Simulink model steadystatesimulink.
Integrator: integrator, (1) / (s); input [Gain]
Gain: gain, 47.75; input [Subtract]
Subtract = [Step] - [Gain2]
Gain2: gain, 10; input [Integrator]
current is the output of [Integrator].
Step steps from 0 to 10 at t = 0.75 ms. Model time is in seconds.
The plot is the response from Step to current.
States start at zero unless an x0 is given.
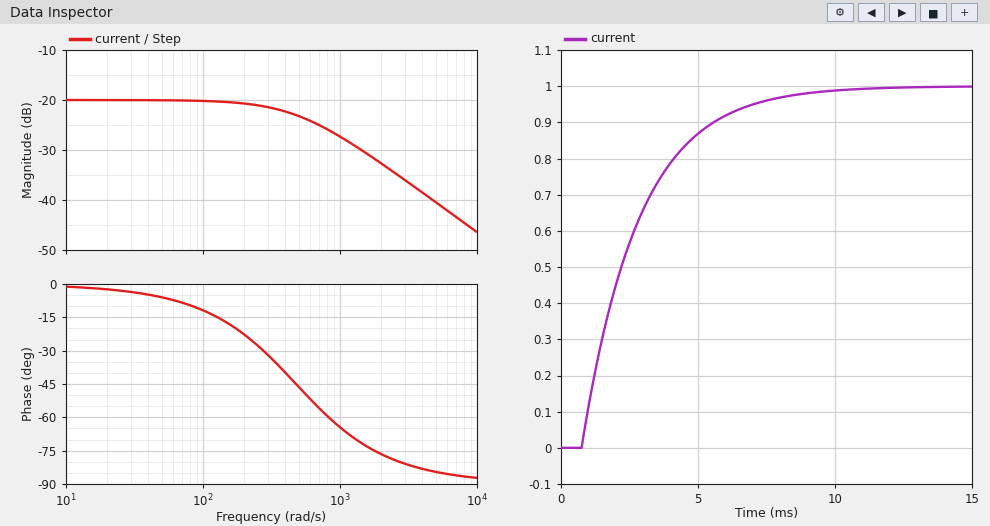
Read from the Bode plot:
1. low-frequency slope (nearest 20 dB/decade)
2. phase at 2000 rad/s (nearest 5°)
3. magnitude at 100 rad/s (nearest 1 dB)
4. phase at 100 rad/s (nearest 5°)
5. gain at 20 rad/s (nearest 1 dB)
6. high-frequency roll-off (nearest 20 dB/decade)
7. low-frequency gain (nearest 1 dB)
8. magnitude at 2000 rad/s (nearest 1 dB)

0 dB/decade
-75°
-20 dB
-10°
-20 dB
-20 dB/decade
-20 dB
-33 dB
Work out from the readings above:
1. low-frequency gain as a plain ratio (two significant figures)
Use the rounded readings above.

0.10
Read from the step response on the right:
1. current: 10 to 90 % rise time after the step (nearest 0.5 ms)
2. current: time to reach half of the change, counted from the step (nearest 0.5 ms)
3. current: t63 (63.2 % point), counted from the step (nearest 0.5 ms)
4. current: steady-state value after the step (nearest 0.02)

4.5 ms
1.5 ms
2.0 ms
1.00
